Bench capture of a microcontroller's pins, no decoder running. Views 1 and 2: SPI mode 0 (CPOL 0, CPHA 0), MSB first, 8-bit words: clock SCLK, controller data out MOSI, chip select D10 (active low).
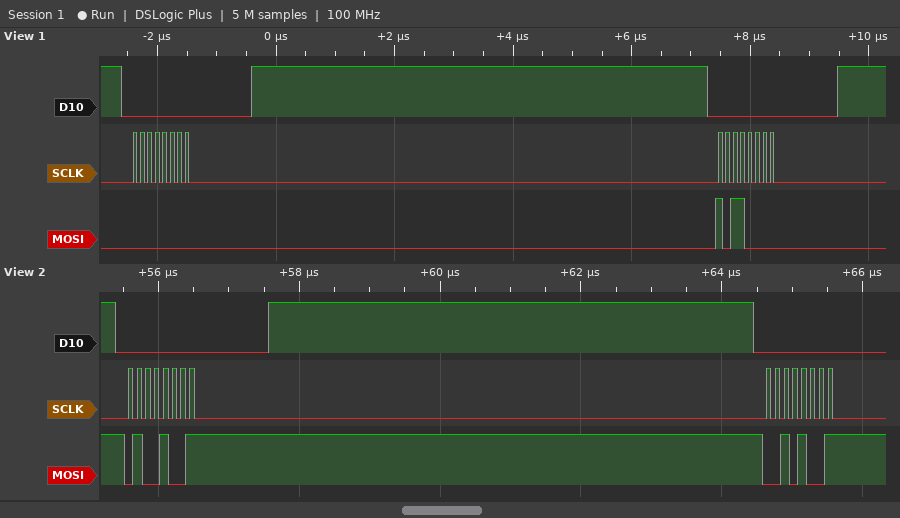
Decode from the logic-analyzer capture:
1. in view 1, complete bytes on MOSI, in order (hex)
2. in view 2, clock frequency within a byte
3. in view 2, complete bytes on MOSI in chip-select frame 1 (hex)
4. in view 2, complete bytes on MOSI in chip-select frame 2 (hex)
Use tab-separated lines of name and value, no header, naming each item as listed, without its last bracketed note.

in view 1, complete bytes on MOSI, in order	00 B0
in view 2, clock frequency within a byte	8 MHz
in view 2, complete bytes on MOSI in chip-select frame 1	49
in view 2, complete bytes on MOSI in chip-select frame 2	29
